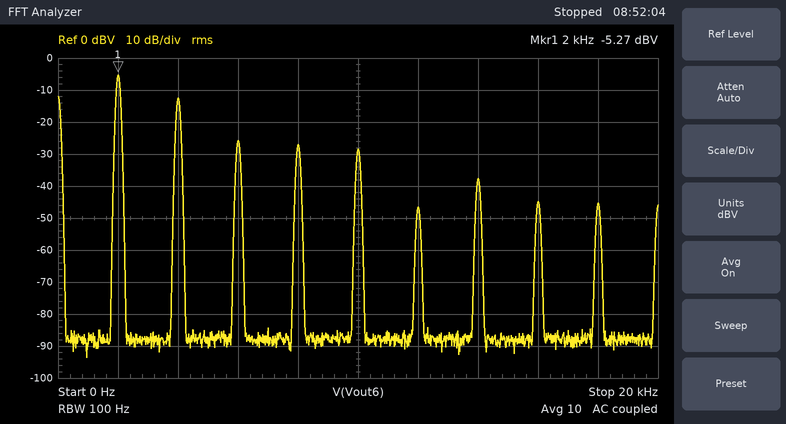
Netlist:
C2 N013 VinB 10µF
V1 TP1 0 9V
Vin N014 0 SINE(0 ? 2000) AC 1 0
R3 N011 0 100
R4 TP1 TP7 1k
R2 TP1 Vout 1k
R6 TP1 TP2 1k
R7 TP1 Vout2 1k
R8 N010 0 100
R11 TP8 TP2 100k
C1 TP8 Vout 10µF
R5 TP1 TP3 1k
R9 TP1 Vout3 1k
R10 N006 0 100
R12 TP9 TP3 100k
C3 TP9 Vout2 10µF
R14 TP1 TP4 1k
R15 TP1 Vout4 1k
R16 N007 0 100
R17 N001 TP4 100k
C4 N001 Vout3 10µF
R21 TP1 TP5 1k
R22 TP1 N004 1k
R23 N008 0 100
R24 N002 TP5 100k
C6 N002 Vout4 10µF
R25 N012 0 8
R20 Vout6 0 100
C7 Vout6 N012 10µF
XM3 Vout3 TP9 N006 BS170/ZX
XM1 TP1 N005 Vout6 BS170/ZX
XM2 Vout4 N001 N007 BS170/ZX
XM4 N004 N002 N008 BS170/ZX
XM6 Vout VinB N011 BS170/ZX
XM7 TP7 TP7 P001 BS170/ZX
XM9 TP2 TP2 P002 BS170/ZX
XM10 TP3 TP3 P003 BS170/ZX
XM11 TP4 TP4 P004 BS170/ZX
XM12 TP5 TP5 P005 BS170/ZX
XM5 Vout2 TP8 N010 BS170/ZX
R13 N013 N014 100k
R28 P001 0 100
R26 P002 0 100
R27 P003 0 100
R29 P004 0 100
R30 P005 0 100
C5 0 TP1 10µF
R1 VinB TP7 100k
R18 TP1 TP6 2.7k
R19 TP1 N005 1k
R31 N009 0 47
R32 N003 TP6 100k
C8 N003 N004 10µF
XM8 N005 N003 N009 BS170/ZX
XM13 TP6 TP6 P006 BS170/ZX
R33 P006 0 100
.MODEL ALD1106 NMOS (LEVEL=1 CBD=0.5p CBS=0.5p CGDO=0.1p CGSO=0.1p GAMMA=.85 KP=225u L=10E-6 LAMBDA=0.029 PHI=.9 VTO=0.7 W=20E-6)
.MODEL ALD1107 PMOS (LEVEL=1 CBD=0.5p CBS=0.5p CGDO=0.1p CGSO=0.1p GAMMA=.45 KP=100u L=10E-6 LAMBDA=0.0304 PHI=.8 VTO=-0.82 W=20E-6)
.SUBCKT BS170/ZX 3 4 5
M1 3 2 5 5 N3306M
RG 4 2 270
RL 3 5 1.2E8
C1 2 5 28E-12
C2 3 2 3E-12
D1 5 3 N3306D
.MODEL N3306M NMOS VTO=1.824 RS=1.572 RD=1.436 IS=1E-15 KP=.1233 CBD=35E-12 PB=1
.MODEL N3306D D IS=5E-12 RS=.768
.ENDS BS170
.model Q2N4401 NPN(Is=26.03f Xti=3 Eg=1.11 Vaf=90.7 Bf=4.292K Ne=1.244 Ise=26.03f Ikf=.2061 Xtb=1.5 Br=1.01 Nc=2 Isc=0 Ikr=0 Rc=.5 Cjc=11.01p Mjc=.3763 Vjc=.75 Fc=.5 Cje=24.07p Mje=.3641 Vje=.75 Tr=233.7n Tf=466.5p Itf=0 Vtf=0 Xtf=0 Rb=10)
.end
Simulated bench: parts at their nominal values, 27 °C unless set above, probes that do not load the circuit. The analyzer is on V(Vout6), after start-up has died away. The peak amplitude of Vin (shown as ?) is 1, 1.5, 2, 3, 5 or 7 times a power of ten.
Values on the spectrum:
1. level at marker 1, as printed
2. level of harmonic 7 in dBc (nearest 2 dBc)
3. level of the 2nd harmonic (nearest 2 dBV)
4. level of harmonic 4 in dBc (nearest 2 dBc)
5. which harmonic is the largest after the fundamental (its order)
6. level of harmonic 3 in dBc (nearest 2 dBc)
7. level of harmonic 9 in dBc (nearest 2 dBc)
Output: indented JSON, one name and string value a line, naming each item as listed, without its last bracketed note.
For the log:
{
  "level at marker 1, as printed": "-5.27 dBV",
  "level of harmonic 7 in dBc": "-32 dBc",
  "level of the 2nd harmonic": "-12 dBV",
  "level of harmonic 4 in dBc": "-22 dBc",
  "which harmonic is the largest after the fundamental": "2",
  "level of harmonic 3 in dBc": "-20 dBc",
  "level of harmonic 9 in dBc": "-40 dBc"
}
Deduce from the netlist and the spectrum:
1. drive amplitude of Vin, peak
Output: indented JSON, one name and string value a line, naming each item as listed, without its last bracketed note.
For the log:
{
  "drive amplitude of Vin, peak": "30 µV"
}
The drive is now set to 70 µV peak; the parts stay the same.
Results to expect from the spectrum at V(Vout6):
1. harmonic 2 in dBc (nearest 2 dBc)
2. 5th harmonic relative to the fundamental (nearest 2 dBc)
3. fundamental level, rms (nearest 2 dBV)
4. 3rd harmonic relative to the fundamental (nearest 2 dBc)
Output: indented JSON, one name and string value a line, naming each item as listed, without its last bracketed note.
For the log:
{
  "harmonic 2 in dBc": "-12 dBc",
  "5th harmonic relative to the fundamental": "-26 dBc",
  "fundamental level, rms": "-6 dBV",
  "3rd harmonic relative to the fundamental": "-14 dBc"
}
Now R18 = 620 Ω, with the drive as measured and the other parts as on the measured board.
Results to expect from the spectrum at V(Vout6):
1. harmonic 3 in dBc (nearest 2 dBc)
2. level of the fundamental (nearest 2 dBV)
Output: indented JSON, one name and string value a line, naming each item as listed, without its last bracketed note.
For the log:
{
  "harmonic 3 in dBc": "-14 dBc",
  "level of the fundamental": "-138 dBV"
}
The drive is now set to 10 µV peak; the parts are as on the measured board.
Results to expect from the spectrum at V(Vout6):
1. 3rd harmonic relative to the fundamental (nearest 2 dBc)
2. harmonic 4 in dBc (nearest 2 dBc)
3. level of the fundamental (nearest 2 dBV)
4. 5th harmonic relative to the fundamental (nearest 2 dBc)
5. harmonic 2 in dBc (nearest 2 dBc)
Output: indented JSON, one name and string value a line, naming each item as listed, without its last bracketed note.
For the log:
{
  "3rd harmonic relative to the fundamental": "-34 dBc",
  "harmonic 4 in dBc": "-28 dBc",
  "level of the fundamental": "-10 dBV",
  "5th harmonic relative to the fundamental": "-44 dBc",
  "harmonic 2 in dBc": "-10 dBc"
}
